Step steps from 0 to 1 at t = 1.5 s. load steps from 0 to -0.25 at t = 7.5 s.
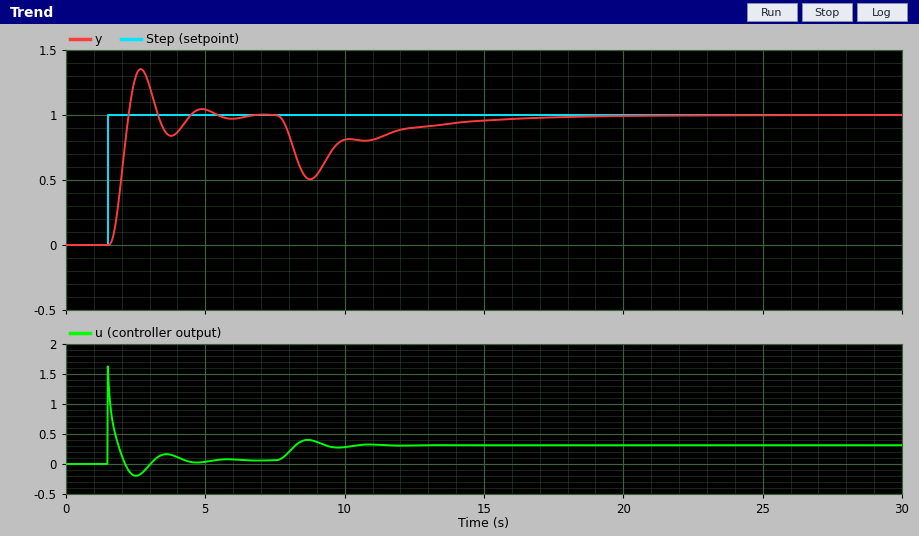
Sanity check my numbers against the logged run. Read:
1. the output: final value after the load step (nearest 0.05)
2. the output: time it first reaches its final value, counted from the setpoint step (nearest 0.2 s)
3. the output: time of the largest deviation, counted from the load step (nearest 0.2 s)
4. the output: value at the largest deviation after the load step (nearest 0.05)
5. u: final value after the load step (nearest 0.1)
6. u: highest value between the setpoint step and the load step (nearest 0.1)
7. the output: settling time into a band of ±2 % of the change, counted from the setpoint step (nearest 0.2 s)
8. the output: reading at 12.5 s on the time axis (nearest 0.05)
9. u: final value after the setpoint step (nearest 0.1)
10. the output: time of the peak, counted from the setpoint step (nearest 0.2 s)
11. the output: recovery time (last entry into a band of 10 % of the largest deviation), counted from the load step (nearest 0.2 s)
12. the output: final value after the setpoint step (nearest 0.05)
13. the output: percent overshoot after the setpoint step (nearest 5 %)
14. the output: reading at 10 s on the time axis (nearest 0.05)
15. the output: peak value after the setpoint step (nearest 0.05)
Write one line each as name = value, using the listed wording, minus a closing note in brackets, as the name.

the output: final value after the load step = 1.00
the output: time it first reaches its final value, counted from the setpoint step = 0.8 s
the output: time of the largest deviation, counted from the load step = 1.2 s
the output: value at the largest deviation after the load step = 0.50
u: final value after the load step = 0.3
u: highest value between the setpoint step and the load step = 1.6
the output: settling time into a band of ±2 % of the change, counted from the setpoint step = 4.8 s
the output: reading at 12.5 s on the time axis = 0.90
u: final value after the setpoint step = 0.1
the output: time of the peak, counted from the setpoint step = 1.2 s
the output: recovery time (last entry into a band of 10 % of the largest deviation), counted from the load step = 7.0 s
the output: final value after the setpoint step = 1.00
the output: percent overshoot after the setpoint step = 35 %
the output: reading at 10 s on the time axis = 0.80
the output: peak value after the setpoint step = 1.35
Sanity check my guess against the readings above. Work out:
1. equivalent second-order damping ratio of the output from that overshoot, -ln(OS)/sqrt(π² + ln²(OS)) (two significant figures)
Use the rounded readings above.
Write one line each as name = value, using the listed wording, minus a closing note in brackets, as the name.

equivalent second-order damping ratio of the output from that overshoot, -ln(OS)/sqrt(π² + ln²(OS)) = 0.32
